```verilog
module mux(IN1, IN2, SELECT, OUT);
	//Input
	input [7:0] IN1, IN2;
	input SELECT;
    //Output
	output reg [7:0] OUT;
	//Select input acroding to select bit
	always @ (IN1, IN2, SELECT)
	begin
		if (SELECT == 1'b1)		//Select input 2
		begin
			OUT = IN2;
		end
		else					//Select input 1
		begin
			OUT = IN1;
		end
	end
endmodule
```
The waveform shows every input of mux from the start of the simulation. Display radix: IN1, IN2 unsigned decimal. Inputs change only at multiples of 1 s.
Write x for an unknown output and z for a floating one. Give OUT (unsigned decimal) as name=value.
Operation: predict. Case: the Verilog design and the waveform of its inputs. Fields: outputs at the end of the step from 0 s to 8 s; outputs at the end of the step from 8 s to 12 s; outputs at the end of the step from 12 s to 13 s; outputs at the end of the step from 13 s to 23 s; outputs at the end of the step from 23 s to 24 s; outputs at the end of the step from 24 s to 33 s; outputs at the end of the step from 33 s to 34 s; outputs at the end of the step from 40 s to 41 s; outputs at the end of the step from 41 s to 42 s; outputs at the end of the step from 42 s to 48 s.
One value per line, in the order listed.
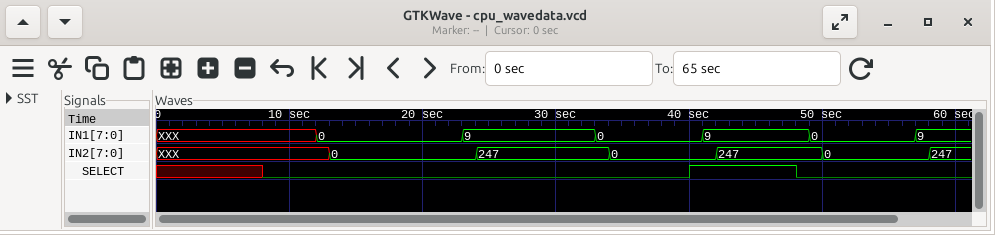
OUT=x
OUT=x
OUT=0
OUT=0
OUT=9
OUT=9
OUT=0
OUT=0
OUT=0
OUT=247
